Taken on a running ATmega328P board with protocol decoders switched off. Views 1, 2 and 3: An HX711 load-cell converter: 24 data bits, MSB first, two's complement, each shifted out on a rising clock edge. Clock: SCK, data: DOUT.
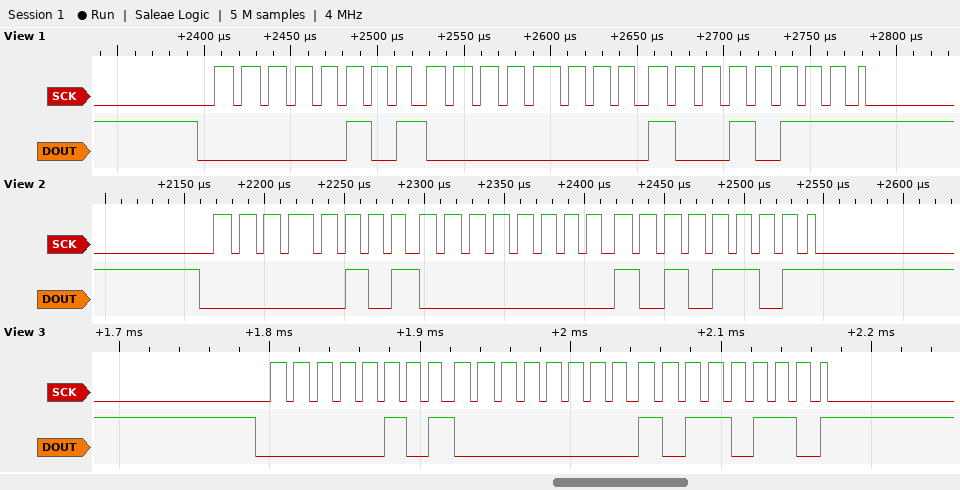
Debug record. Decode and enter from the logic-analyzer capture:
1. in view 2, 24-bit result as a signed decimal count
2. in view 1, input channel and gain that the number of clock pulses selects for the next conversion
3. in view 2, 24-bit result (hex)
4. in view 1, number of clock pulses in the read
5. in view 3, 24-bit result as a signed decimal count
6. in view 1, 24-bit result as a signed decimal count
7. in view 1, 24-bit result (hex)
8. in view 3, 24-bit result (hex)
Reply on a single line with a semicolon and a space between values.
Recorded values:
327853; channel A, gain 128; 0x0500AD; 25; 327862; 327831; 0x050097; 0x0500B6
